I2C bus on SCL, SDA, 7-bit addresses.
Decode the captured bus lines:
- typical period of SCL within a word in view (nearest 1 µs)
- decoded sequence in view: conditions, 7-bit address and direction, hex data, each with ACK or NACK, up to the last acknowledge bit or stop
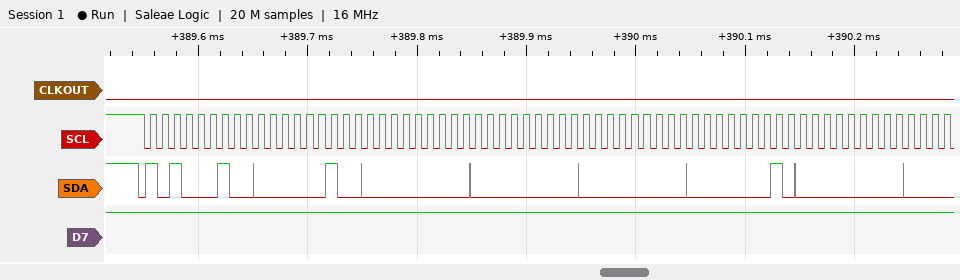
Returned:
11 µs
start, address 51 write ACK, 02 ACK, 00 ACK, 00 ACK, 00 ACK, 01 ACK, 00 ACK
